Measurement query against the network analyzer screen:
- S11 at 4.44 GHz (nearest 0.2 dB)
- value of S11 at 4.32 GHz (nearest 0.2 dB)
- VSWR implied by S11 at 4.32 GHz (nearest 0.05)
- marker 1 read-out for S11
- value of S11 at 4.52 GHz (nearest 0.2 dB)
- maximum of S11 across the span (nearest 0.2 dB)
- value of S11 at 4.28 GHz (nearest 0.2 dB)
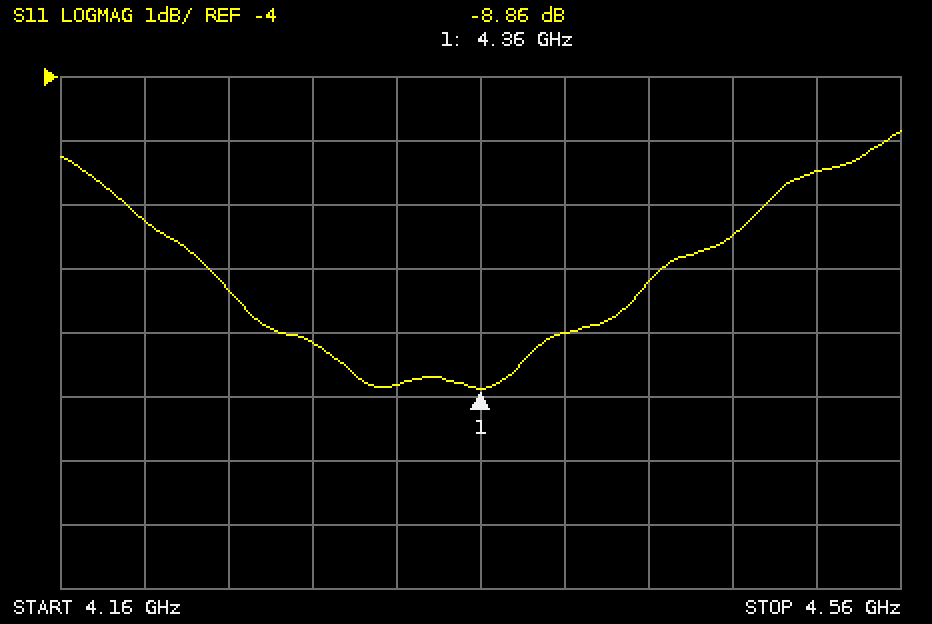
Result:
-7.2 dB
-8.8 dB
2.15
-8.86 dB
-5.4 dB
-4.8 dB
-8.2 dB
